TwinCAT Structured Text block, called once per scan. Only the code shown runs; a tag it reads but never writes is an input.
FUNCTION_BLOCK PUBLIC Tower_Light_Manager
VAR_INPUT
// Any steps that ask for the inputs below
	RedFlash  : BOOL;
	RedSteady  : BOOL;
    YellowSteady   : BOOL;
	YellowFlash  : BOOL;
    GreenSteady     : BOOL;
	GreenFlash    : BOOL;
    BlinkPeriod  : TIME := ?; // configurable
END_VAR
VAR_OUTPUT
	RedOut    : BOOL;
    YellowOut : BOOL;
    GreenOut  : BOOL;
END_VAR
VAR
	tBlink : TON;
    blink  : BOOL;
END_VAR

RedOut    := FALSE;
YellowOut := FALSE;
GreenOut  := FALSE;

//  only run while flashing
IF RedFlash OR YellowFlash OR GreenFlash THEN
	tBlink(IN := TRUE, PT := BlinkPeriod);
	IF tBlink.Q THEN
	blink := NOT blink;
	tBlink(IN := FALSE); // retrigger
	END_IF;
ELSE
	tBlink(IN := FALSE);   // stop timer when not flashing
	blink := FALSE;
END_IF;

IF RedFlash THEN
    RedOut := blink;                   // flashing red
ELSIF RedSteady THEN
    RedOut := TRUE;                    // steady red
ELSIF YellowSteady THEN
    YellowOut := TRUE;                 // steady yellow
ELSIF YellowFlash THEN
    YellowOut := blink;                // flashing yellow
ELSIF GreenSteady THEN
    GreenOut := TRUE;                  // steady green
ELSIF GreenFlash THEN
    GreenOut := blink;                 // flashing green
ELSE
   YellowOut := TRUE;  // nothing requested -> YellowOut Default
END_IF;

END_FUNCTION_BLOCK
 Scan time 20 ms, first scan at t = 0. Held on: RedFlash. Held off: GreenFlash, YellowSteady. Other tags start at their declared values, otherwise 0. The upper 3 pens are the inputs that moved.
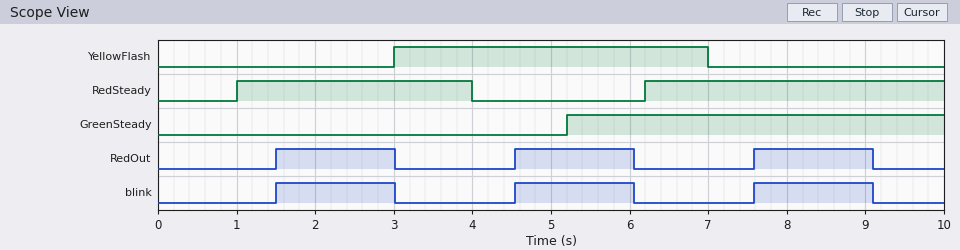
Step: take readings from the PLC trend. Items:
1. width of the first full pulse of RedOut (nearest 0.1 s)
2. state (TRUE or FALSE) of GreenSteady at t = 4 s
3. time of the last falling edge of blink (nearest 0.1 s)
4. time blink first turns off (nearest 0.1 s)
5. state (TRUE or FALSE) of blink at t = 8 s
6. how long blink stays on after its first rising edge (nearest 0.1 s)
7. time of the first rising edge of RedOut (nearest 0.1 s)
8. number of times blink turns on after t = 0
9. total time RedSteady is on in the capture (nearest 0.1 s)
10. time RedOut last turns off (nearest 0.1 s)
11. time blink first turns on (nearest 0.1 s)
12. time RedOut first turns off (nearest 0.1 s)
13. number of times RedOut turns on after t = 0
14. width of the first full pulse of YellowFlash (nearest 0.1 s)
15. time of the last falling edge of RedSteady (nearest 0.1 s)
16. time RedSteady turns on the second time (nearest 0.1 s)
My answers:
1.5 s
FALSE
9.1 s
3.0 s
TRUE
1.5 s
1.5 s
3
6.8 s
9.1 s
1.5 s
3.0 s
3
4.0 s
4.0 s
6.2 s
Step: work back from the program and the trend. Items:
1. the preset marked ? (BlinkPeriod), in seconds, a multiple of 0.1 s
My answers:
1.5 s
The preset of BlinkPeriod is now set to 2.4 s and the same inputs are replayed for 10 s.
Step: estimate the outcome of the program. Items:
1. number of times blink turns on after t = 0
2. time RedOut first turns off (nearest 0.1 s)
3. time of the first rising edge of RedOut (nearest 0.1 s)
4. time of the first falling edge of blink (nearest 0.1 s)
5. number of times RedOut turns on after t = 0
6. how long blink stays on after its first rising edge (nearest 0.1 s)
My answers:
2
4.8 s
2.4 s
4.8 s
2
2.4 s
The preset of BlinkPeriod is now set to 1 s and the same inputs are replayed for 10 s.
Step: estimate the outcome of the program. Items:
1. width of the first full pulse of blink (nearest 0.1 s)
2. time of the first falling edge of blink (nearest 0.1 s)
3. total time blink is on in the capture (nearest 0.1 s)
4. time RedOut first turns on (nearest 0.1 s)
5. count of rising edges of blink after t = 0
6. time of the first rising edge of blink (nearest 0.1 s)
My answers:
1.0 s
2.0 s
4.9 s
1.0 s
5
1.0 s
